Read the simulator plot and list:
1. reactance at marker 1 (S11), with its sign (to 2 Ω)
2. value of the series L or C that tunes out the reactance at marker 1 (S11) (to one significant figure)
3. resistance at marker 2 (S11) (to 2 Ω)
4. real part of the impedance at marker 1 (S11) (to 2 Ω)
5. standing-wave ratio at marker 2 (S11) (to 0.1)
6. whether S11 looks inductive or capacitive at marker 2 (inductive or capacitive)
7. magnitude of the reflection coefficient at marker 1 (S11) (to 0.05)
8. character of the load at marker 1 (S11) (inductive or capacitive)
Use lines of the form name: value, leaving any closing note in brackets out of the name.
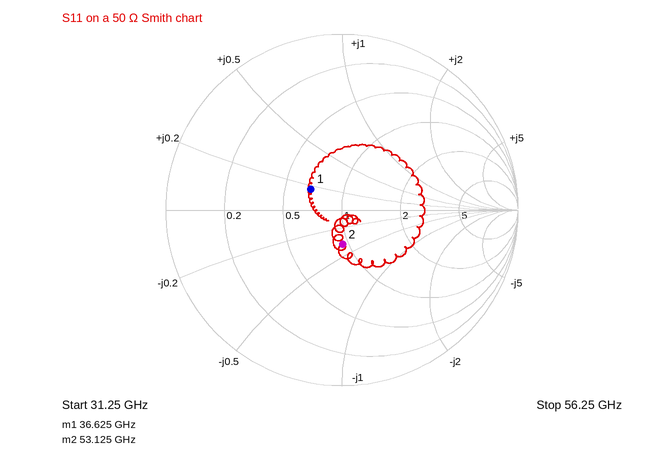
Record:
reactance at marker 1 (S11), with its sign: +8 Ω
value of the series L or C that tunes out the reactance at marker 1 (S11): 500 fF
resistance at marker 2 (S11): 46 Ω
real part of the impedance at marker 1 (S11): 34 Ω
standing-wave ratio at marker 2 (S11): 1.5
whether S11 looks inductive or capacitive at marker 2: capacitive
magnitude of the reflection coefficient at marker 1 (S11): 0.20
character of the load at marker 1 (S11): inductive
